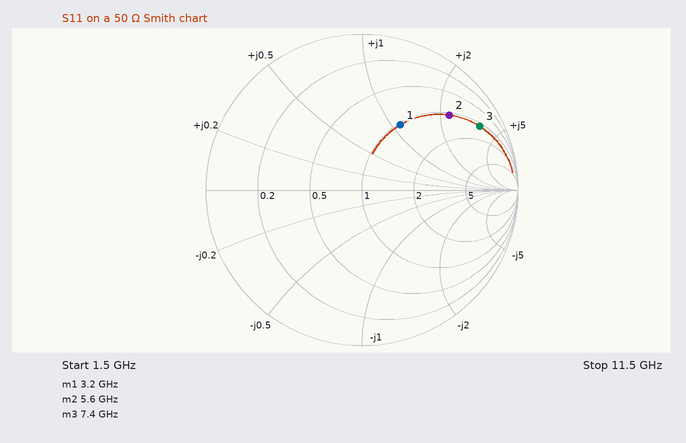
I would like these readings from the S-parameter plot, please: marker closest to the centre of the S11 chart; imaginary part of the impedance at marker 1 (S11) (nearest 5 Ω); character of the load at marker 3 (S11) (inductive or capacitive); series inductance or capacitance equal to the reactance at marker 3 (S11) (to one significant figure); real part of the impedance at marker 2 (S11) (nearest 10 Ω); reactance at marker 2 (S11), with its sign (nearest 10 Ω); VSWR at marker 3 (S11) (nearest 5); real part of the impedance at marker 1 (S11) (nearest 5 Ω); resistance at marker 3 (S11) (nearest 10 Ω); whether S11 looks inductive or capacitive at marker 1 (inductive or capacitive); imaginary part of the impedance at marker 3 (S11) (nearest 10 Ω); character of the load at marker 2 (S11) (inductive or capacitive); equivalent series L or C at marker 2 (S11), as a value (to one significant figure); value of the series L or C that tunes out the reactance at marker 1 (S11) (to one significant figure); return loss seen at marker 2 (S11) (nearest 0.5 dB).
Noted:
marker 1
+55 Ω
inductive
4 nH
50 Ω
+110 Ω
15
50 Ω
60 Ω
inductive
+180 Ω
inductive
3 nH
900 fF
2.5 dB
